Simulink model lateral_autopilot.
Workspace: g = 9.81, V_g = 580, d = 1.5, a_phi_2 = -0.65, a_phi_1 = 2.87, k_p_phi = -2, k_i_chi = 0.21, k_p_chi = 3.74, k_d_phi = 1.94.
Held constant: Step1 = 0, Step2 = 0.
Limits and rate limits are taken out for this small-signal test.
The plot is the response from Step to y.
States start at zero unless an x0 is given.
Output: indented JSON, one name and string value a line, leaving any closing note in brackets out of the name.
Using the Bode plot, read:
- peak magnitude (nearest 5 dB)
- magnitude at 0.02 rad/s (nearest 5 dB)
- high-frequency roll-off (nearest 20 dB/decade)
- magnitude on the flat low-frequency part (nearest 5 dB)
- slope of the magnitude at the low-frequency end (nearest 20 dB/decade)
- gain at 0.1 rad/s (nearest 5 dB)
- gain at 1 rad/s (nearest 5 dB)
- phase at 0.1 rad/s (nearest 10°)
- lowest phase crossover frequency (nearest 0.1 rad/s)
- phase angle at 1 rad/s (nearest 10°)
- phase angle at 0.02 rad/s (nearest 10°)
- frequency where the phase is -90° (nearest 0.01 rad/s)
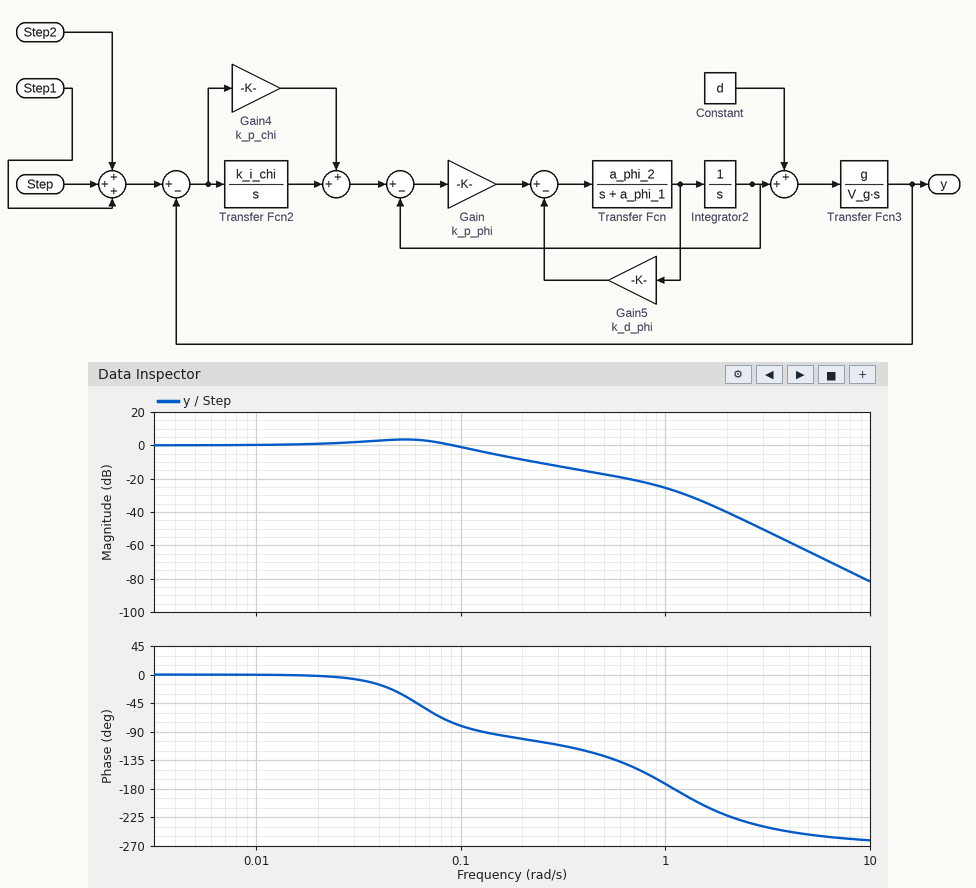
{
  "peak magnitude": "5 dB",
  "magnitude at 0.02 rad/s": "0 dB",
  "high-frequency roll-off": "-60 dB/decade",
  "magnitude on the flat low-frequency part": "0 dB",
  "slope of the magnitude at the low-frequency end": "0 dB/decade",
  "gain at 0.1 rad/s": "0 dB",
  "gain at 1 rad/s": "-25 dB",
  "phase at 0.1 rad/s": "-80°",
  "lowest phase crossover frequency": "1.1 rad/s",
  "phase angle at 1 rad/s": "-170°",
  "phase angle at 0.02 rad/s": "0°",
  "frequency where the phase is -90°": "0.13 rad/s"
}
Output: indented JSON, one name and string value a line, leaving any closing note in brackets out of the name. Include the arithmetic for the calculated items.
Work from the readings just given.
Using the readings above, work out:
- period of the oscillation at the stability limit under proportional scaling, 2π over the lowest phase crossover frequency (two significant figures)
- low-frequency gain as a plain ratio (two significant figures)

{
  "period of the oscillation at the stability limit under proportional scaling, 2π over the lowest phase crossover frequency": "2π / 1.1 = 5.7 s",
  "low-frequency gain as a plain ratio": "10^(0 / 20) = 1.0"
}
